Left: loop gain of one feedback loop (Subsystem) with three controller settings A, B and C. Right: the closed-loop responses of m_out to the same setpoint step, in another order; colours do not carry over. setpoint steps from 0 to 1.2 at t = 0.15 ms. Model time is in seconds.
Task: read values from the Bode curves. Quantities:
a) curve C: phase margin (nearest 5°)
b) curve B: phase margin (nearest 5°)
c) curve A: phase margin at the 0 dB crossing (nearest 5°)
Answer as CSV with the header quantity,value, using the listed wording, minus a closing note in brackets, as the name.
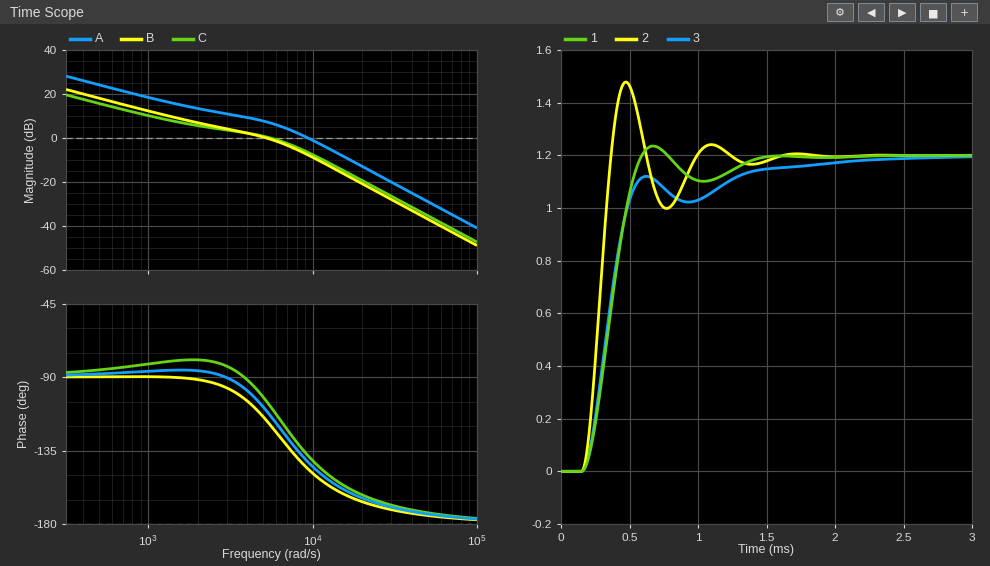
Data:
quantity,value
curve C: phase margin,70°
curve B: phase margin,65°
curve A: phase margin at the 0 dB crossing,40°
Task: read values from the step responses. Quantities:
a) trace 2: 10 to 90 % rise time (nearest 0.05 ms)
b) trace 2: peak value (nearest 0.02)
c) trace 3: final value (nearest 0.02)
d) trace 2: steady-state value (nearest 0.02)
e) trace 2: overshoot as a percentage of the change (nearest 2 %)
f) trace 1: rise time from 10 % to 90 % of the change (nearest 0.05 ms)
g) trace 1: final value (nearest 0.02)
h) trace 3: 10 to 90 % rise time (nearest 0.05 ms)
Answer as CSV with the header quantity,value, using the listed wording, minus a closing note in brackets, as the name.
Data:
quantity,value
trace 2: 10 to 90 % rise time,0.15 ms
trace 2: peak value,1.48
trace 3: final value,1.20
trace 2: steady-state value,1.20
trace 2: overshoot as a percentage of the change,24 %
trace 1: rise time from 10 % to 90 % of the change,0.30 ms
trace 1: final value,1.20
trace 3: 10 to 90 % rise time,0.30 ms
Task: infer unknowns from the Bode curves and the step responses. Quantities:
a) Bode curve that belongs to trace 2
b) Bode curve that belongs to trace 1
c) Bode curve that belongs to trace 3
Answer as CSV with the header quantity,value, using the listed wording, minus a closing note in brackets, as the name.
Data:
quantity,value
Bode curve that belongs to trace 2,A
Bode curve that belongs to trace 1,B
Bode curve that belongs to trace 3,C
